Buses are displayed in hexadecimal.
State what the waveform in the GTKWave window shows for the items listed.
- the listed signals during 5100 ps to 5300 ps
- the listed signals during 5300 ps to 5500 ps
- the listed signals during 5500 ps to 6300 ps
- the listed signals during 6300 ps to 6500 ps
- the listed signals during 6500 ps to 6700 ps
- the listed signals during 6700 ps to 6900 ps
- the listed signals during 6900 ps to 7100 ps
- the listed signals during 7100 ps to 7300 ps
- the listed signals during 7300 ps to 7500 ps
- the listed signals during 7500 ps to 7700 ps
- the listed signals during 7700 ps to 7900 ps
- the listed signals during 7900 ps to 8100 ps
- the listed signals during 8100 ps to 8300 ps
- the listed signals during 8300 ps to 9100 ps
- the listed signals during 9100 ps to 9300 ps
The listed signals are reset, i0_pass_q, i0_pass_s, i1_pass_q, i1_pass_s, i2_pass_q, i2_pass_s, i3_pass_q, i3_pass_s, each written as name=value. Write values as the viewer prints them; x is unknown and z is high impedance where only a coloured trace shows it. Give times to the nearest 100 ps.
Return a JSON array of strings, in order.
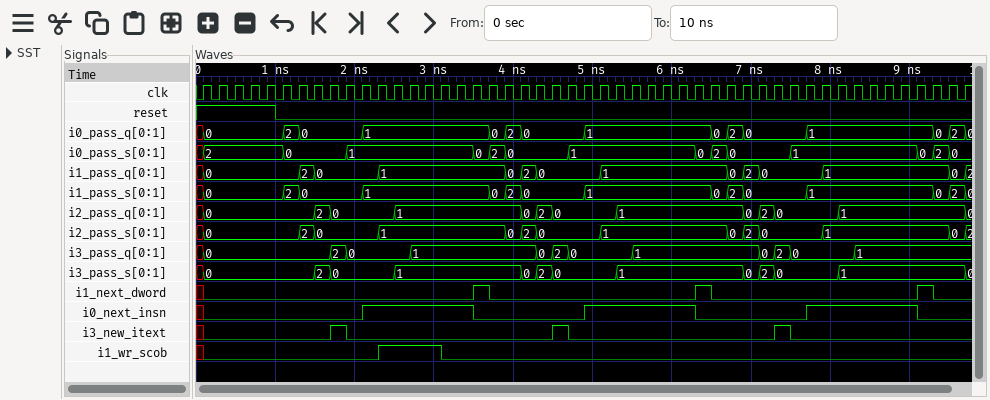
["reset=0, i0_pass_q=1, i0_pass_s=1, i1_pass_q=1, i1_pass_s=1, i2_pass_q=0, i2_pass_s=1, i3_pass_q=0, i3_pass_s=0", "reset=0, i0_pass_q=1, i0_pass_s=1, i1_pass_q=1, i1_pass_s=1, i2_pass_q=1, i2_pass_s=1, i3_pass_q=0, i3_pass_s=1", "reset=0, i0_pass_q=1, i0_pass_s=1, i1_pass_q=1, i1_pass_s=1, i2_pass_q=1, i2_pass_s=1, i3_pass_q=1, i3_pass_s=1", "reset=0, i0_pass_q=1, i0_pass_s=0, i1_pass_q=1, i1_pass_s=1, i2_pass_q=1, i2_pass_s=1, i3_pass_q=1, i3_pass_s=1", "reset=0, i0_pass_q=0, i0_pass_s=2, i1_pass_q=1, i1_pass_s=0, i2_pass_q=1, i2_pass_s=1, i3_pass_q=1, i3_pass_s=1", "reset=0, i0_pass_q=2, i0_pass_s=0, i1_pass_q=0, i1_pass_s=2, i2_pass_q=1, i2_pass_s=0, i3_pass_q=1, i3_pass_s=1", "reset=0, i0_pass_q=0, i0_pass_s=0, i1_pass_q=2, i1_pass_s=0, i2_pass_q=0, i2_pass_s=2, i3_pass_q=1, i3_pass_s=0", "reset=0, i0_pass_q=0, i0_pass_s=0, i1_pass_q=0, i1_pass_s=0, i2_pass_q=2, i2_pass_s=0, i3_pass_q=0, i3_pass_s=2", "reset=0, i0_pass_q=0, i0_pass_s=0, i1_pass_q=0, i1_pass_s=0, i2_pass_q=0, i2_pass_s=0, i3_pass_q=2, i3_pass_s=0", "reset=0, i0_pass_q=0, i0_pass_s=1, i1_pass_q=0, i1_pass_s=0, i2_pass_q=0, i2_pass_s=0, i3_pass_q=0, i3_pass_s=0", "reset=0, i0_pass_q=1, i0_pass_s=1, i1_pass_q=0, i1_pass_s=1, i2_pass_q=0, i2_pass_s=0, i3_pass_q=0, i3_pass_s=0", "reset=0, i0_pass_q=1, i0_pass_s=1, i1_pass_q=1, i1_pass_s=1, i2_pass_q=0, i2_pass_s=1, i3_pass_q=0, i3_pass_s=0", "reset=0, i0_pass_q=1, i0_pass_s=1, i1_pass_q=1, i1_pass_s=1, i2_pass_q=1, i2_pass_s=1, i3_pass_q=0, i3_pass_s=1", "reset=0, i0_pass_q=1, i0_pass_s=1, i1_pass_q=1, i1_pass_s=1, i2_pass_q=1, i2_pass_s=1, i3_pass_q=1, i3_pass_s=1", "reset=0, i0_pass_q=1, i0_pass_s=0, i1_pass_q=1, i1_pass_s=1, i2_pass_q=1, i2_pass_s=1, i3_pass_q=1, i3_pass_s=1"]
